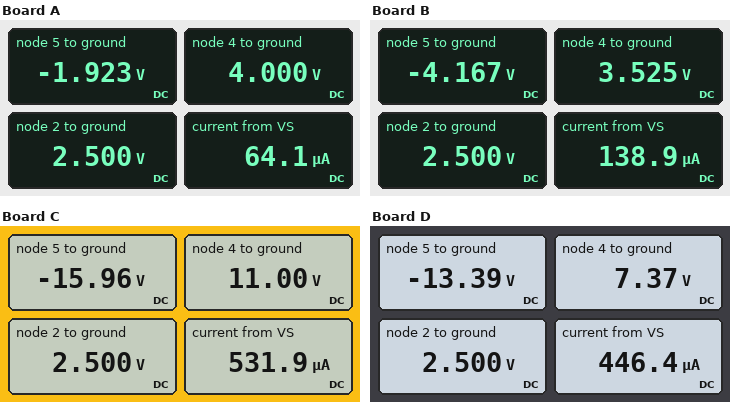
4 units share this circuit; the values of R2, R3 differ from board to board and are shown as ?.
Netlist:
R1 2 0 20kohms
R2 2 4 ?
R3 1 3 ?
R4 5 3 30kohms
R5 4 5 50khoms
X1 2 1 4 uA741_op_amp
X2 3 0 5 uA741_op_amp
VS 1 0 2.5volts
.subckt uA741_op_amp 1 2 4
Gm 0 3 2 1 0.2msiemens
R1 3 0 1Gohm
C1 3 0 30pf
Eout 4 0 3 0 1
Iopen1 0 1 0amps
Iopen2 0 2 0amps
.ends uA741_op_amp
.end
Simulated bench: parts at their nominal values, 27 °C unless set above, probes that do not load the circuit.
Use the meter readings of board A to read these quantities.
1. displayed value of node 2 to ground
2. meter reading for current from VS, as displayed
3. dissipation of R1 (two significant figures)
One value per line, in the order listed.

2.500 V
64.1 µA
310 µW
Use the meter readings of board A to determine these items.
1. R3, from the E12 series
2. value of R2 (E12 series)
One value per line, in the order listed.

39 kΩ
12 kΩ
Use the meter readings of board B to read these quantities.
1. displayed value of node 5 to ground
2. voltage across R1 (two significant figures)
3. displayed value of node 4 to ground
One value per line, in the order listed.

-4.167 V
2.5 V
3.525 V
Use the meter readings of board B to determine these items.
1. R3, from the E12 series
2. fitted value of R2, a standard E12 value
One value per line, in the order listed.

18 kΩ
8.2 kΩ
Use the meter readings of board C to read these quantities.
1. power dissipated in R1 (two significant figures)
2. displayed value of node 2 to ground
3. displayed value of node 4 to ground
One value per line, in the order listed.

310 µW
2.500 V
11.00 V
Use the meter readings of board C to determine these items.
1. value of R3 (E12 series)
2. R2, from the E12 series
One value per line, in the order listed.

4.7 kΩ
68 kΩ
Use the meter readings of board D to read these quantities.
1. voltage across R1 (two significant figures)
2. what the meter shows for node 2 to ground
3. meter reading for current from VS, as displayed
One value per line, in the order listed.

2.5 V
2.500 V
446.4 µA
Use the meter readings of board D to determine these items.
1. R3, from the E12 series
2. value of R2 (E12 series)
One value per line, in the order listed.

5.6 kΩ
39 kΩ
